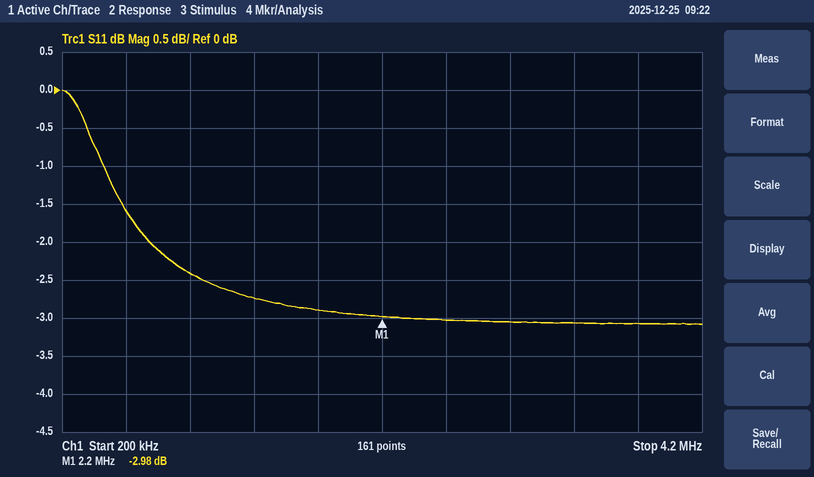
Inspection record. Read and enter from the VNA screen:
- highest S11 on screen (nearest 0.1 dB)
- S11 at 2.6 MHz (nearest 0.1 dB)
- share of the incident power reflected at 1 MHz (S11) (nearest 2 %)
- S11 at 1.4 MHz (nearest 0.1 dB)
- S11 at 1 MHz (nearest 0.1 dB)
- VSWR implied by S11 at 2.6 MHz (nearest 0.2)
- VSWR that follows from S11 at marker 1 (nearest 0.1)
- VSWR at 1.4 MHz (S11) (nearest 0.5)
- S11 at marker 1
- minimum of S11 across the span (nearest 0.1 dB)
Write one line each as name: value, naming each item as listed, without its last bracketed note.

highest S11 on screen: 0.0 dB
S11 at 2.6 MHz: -3.0 dB
share of the incident power reflected at 1 MHz (S11): 58 %
S11 at 1.4 MHz: -2.7 dB
S11 at 1 MHz: -2.4 dB
VSWR implied by S11 at 2.6 MHz: 5.8
VSWR that follows from S11 at marker 1: 5.9
VSWR at 1.4 MHz (S11): 6.5
S11 at marker 1: -2.98 dB
minimum of S11 across the span: -3.1 dB
